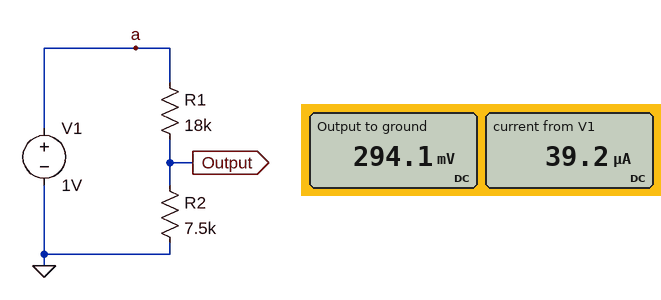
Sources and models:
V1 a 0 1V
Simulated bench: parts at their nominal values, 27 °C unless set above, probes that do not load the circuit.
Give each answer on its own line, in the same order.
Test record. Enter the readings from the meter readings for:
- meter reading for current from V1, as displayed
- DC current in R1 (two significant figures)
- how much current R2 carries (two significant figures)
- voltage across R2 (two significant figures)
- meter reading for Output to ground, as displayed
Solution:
39.2 µA
39 µA
39 µA
290 mV
294.1 mV
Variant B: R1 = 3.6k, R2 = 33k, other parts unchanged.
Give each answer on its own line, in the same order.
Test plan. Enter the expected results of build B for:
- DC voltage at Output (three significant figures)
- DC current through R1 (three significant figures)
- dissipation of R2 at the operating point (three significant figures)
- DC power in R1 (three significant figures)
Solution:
902 mV
27.3 µA
24.6 µW
2.69 µW
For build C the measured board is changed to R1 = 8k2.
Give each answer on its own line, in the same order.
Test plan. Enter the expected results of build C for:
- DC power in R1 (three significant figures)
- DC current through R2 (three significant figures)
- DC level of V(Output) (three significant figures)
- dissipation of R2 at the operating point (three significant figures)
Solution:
33.3 µW
63.7 µA
478 mV
30.4 µW
